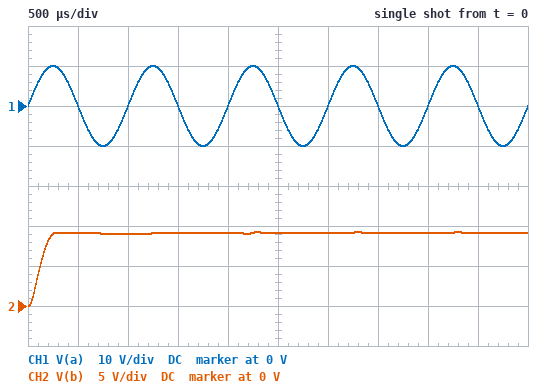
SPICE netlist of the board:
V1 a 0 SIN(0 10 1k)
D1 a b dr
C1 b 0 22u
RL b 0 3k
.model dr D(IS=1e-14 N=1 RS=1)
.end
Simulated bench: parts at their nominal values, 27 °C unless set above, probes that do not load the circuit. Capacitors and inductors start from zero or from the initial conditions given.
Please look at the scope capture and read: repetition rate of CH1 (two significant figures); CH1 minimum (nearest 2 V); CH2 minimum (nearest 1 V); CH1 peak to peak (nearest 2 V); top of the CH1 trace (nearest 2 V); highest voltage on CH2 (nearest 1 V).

1.0 kHz
-10 V
0 V
20 V
10 V
9 V
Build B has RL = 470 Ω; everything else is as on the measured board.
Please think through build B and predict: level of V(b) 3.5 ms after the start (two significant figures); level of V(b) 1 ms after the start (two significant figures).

8.9 V
8.5 V
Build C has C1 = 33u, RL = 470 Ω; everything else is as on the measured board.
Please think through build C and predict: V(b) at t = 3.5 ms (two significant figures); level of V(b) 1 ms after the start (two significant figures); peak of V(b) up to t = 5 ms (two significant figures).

8.9 V
8.6 V
9.1 V
